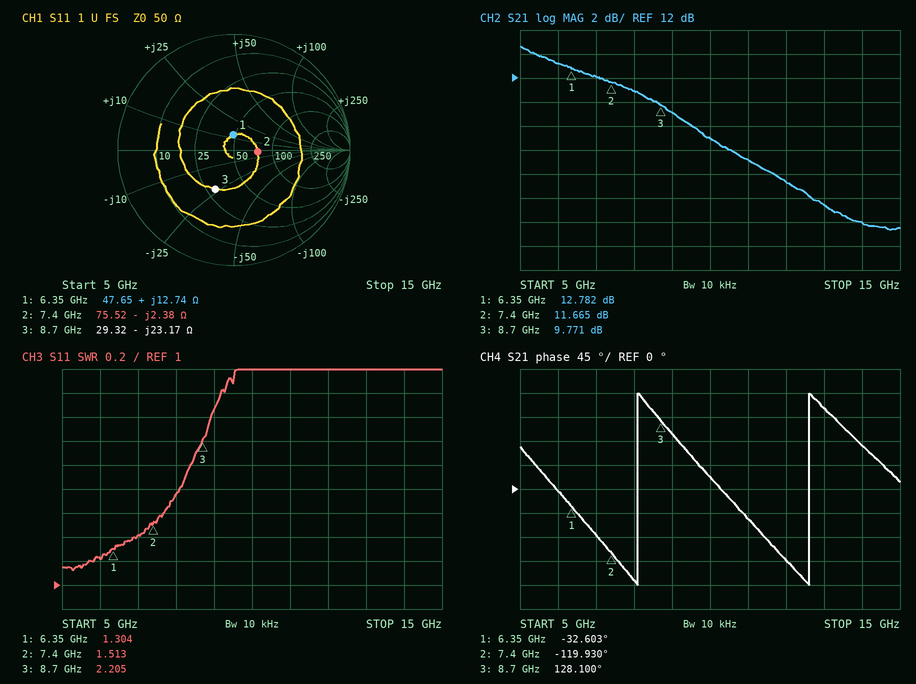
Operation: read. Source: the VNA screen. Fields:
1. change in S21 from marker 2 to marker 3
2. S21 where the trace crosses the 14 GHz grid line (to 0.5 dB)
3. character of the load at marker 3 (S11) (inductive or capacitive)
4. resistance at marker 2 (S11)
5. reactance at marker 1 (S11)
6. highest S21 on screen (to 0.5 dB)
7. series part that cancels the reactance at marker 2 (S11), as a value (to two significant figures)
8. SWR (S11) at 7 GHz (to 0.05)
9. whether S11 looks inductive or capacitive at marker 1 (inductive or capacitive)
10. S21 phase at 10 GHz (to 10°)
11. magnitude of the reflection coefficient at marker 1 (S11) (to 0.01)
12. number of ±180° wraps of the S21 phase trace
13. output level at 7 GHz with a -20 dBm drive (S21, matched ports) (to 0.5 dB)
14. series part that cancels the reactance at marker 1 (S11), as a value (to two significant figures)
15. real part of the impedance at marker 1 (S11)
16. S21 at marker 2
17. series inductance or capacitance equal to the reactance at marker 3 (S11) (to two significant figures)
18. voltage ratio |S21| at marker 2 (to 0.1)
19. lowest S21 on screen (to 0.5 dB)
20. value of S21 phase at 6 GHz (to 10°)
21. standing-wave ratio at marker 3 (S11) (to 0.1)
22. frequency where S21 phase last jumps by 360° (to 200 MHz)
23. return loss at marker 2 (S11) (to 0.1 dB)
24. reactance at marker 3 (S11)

-1.894 dB
0.0 dB
capacitive
75.52 Ω
+12.74 Ω
14.5 dB
51 pH
1.40
inductive
20°
0.13
2
-8.0 dBm
2.0 pF
47.65 Ω
11.665 dB
790 fF
3.8
-0.5 dB
0°
2.2
12.6 GHz
13.8 dB
-23.17 Ω
